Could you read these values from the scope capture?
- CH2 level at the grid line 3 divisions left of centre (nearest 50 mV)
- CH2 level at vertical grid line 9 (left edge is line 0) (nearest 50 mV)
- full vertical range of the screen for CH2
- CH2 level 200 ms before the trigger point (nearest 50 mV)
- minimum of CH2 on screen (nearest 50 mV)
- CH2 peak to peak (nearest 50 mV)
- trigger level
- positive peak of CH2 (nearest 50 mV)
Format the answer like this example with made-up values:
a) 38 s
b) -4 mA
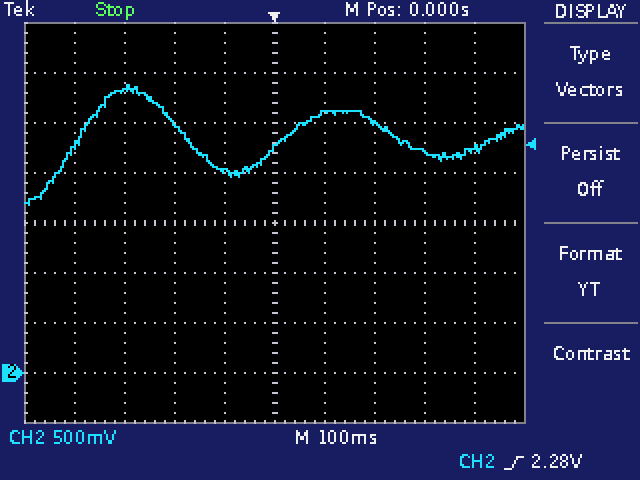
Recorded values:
a) 2.85 V
b) 2.25 V
c) 4 V
d) 2.50 V
e) 1.70 V
f) 1.20 V
g) 2.28 V
h) 2.90 V
